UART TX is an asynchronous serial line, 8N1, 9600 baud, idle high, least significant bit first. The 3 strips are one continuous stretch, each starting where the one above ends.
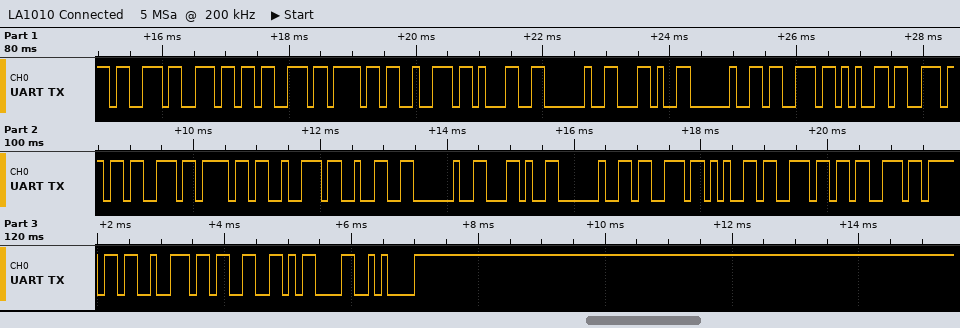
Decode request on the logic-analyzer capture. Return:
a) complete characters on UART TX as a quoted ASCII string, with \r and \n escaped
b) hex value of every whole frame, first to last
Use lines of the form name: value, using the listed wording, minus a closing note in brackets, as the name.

complete characters on UART TX as a quoted ASCII string, with \r and \n escaped: "snsor1 , sensor2 , sensor3\r\n"
hex value of every whole frame, first to last: 73 6E 73 6F 72 31 20 2C 20 73 65 6E 73 6F 72 32 20 2C 20 73 65 6E 73 6F 72 33 0D 0A
